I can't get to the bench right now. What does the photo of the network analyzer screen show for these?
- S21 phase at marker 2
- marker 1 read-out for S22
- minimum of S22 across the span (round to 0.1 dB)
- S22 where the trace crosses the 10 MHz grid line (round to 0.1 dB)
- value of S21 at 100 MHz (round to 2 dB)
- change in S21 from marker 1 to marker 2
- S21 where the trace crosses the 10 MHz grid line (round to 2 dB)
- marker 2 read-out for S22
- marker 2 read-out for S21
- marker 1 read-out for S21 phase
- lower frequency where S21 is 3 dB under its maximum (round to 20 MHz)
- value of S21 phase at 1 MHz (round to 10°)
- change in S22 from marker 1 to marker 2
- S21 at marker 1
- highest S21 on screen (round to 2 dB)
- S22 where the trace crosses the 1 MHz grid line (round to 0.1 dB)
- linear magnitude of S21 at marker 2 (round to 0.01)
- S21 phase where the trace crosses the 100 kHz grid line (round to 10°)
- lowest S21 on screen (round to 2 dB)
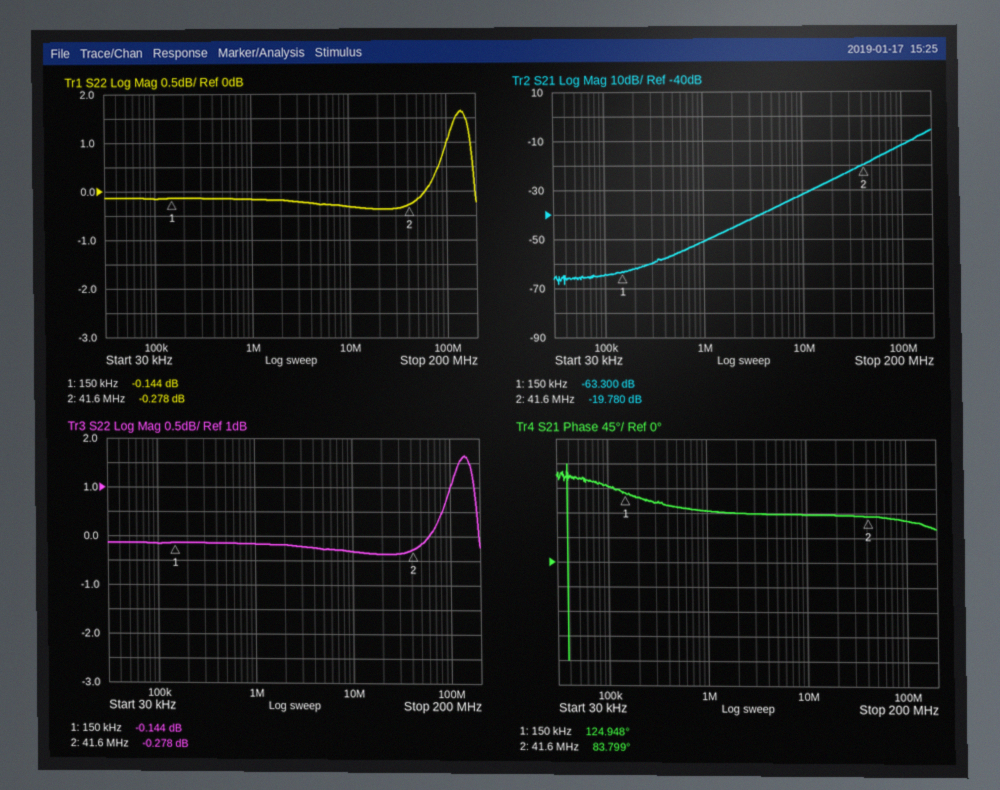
83.799°
-0.144 dB
-0.4 dB
-0.3 dB
-12 dB
43.520 dB
-32 dB
-0.278 dB
-19.780 dB
124.948°
140 MHz
90°
-0.134 dB
-63.300 dB
-6 dB
-0.2 dB
0.10
140°
-68 dB
